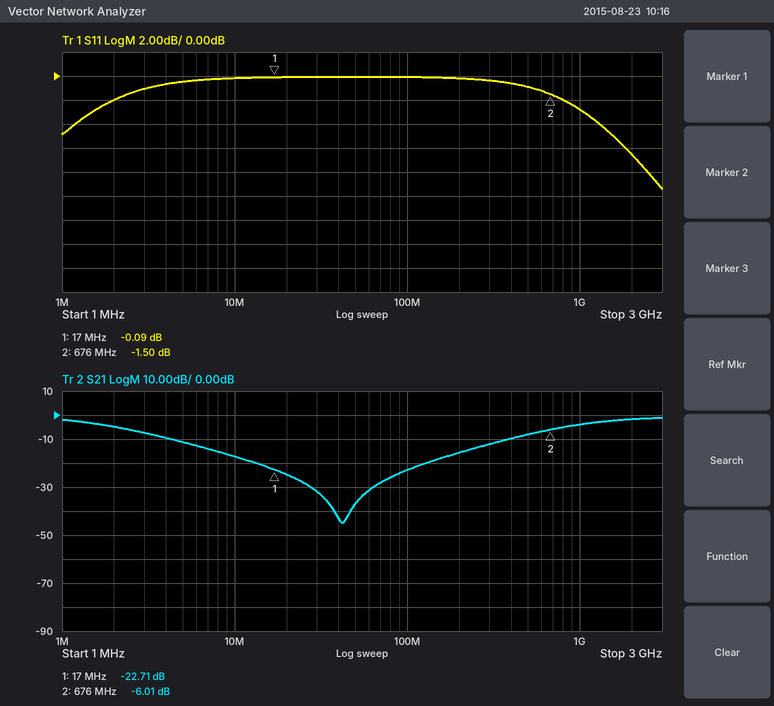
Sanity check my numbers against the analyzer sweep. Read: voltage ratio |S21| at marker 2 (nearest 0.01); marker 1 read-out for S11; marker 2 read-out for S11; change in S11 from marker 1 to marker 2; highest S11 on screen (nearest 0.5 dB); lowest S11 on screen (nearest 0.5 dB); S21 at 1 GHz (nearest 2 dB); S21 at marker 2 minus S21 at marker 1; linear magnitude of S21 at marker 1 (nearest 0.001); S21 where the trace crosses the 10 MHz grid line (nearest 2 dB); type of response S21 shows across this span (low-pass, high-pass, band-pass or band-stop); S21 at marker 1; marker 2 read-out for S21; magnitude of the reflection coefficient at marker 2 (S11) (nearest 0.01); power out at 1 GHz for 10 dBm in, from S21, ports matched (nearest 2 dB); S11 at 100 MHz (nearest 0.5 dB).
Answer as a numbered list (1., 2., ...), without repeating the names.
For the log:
1. 0.50
2. -0.09 dB
3. -1.50 dB
4. -1.41 dB
5. 0.0 dB
6. -9.5 dB
7. -4 dB
8. 16.70 dB
9. 0.073
10. -18 dB
11. band-stop
12. -22.71 dB
13. -6.01 dB
14. 0.84
15. 6 dBm
16. 0.0 dB
